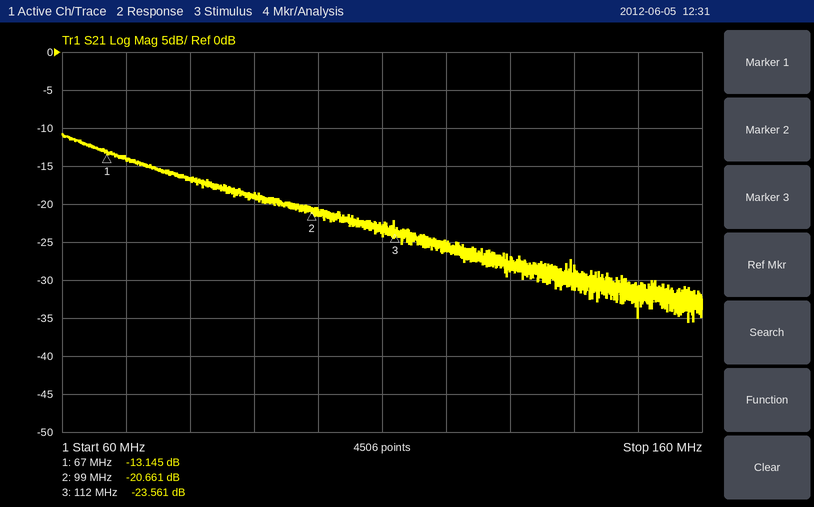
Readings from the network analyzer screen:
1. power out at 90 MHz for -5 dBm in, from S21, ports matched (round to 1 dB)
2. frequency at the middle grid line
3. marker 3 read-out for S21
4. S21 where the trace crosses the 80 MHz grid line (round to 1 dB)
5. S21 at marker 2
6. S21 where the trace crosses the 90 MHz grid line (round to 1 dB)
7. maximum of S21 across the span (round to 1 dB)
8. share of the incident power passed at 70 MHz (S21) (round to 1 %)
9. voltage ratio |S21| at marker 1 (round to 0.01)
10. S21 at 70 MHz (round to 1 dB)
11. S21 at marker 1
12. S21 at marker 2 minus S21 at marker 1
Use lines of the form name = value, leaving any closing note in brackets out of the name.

power out at 90 MHz for -5 dBm in, from S21, ports matched = -24 dBm
frequency at the middle grid line = 110 MHz
marker 3 read-out for S21 = -23.561 dB
S21 where the trace crosses the 80 MHz grid line = -17 dB
S21 at marker 2 = -20.661 dB
S21 where the trace crosses the 90 MHz grid line = -19 dB
maximum of S21 across the span = -11 dB
share of the incident power passed at 70 MHz (S21) = 4 %
voltage ratio |S21| at marker 1 = 0.22
S21 at 70 MHz = -14 dB
S21 at marker 1 = -13.145 dB
S21 at marker 2 minus S21 at marker 1 = -7.516 dB
